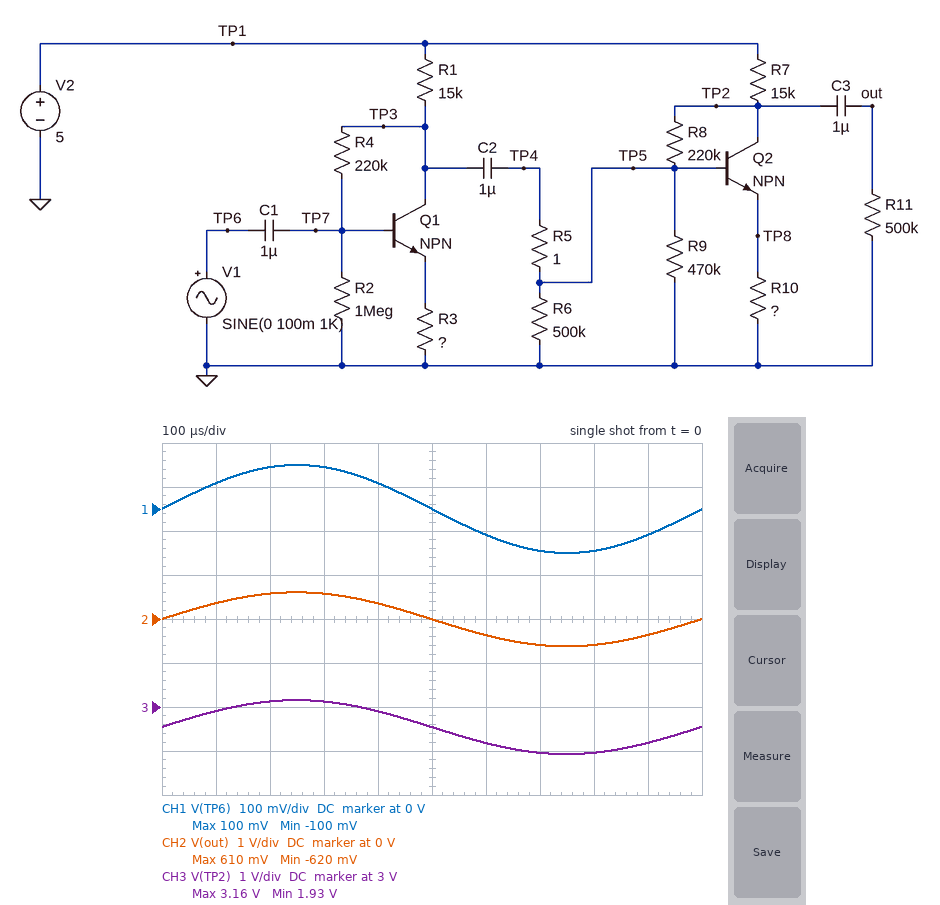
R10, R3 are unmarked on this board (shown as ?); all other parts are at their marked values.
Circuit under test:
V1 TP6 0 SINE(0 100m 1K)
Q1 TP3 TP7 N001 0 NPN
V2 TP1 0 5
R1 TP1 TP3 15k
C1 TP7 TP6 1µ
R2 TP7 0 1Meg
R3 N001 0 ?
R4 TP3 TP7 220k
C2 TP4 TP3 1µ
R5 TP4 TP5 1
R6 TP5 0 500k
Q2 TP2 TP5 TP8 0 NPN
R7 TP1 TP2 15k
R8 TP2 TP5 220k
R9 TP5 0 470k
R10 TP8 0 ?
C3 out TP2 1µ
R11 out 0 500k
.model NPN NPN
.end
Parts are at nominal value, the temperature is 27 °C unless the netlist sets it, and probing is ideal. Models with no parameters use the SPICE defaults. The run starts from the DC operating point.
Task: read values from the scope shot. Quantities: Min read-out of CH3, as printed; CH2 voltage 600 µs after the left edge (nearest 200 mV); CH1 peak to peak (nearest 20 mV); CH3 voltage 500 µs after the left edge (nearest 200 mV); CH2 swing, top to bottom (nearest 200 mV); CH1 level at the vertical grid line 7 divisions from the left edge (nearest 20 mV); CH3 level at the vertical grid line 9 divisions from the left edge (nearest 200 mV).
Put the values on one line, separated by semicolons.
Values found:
1.93 V; -400 mV; 200 mV; 2.6 V; 1.2 V; -100 mV; 2.2 V
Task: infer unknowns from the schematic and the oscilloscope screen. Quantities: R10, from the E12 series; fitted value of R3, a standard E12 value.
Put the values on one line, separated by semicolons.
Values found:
2.7 kΩ; 6.8 kΩ
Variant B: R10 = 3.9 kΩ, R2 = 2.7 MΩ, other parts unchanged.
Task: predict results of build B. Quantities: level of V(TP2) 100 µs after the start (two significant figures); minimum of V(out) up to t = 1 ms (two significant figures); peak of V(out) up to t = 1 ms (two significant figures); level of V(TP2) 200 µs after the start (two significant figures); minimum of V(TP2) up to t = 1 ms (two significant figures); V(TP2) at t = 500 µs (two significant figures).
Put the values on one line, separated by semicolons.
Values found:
3.0 V; -470 mV; 460 mV; 3.2 V; 2.3 V; 2.8 V
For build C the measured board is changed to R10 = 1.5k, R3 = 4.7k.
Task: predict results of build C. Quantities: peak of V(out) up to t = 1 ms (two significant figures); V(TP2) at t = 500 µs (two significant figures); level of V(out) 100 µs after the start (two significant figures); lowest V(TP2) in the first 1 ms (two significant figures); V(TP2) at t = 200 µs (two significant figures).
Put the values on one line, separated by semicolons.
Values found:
1.3 V; 2.3 V; 770 mV; 940 mV; 3.5 V
